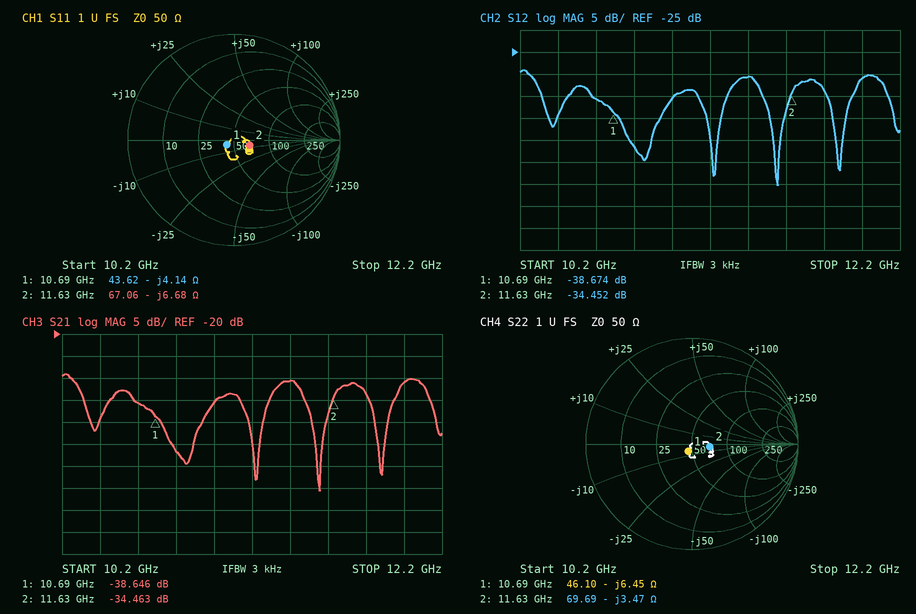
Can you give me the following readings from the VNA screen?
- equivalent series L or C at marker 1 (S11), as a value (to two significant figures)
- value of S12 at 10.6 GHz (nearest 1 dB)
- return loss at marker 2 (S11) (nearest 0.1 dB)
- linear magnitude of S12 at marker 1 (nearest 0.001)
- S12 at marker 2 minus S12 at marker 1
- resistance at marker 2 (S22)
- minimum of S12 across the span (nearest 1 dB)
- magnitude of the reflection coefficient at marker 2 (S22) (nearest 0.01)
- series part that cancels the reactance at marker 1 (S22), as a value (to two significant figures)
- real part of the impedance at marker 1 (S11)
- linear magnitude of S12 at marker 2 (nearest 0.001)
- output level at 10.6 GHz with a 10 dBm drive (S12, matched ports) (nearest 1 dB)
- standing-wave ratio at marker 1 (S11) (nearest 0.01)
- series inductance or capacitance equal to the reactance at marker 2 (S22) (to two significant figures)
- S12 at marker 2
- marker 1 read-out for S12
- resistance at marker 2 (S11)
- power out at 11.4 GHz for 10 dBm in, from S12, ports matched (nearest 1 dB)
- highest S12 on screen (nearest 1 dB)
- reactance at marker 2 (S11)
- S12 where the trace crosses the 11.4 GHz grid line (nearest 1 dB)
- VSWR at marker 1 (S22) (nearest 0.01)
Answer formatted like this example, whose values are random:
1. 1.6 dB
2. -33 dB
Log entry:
1. 3.6 pF
2. -36 dB
3. 16.1 dB
4. 0.012
5. 4.222 dB
6. 69.69 Ω
7. -55 dB
8. 0.17
9. 96 pH
10. 43.62 Ω
11. 0.019
12. -26 dBm
13. 1.18
14. 3.9 pF
15. -34.452 dB
16. -38.674 dB
17. 67.06 Ω
18. -21 dBm
19. -29 dB
20. -6.68 Ω
21. -31 dB
22. 1.17
